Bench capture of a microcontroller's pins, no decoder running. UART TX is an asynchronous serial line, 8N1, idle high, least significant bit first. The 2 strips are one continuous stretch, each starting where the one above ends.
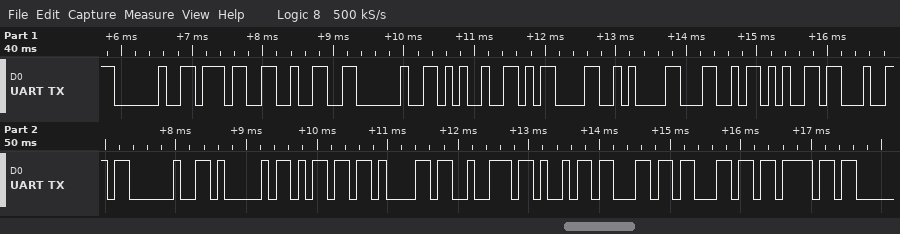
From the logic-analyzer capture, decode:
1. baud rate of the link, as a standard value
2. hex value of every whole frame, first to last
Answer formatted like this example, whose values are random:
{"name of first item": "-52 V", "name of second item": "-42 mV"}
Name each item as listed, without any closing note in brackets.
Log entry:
{"baud rate of the link, as a standard value": "9600 baud", "hex value of every whole frame, first to last": "0x20 0x37 0x32 0x20 0x25 0x0D 0x0A 0x4C 0x65 0x64 0x20 0x41 0x6D 0x61 0x72 0x69 0x6C 0x6C 0x6F"}
